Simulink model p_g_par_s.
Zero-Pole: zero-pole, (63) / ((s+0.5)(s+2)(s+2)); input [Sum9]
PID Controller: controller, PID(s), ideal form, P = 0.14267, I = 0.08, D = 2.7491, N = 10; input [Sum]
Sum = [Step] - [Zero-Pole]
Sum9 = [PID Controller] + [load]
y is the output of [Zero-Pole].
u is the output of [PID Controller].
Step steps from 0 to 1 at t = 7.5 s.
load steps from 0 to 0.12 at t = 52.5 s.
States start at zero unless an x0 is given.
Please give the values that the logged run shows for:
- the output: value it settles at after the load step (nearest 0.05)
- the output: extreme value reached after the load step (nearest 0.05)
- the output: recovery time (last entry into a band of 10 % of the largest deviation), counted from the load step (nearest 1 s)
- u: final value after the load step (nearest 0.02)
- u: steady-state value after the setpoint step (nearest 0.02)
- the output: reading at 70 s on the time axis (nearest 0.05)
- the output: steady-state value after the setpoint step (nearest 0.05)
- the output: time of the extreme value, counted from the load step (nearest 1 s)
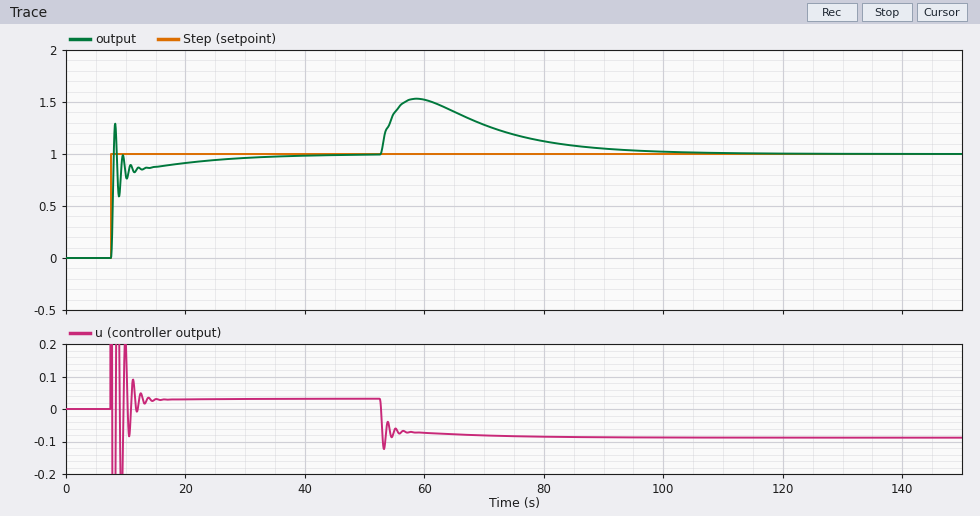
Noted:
1.00
1.55
37 s
-0.08
0.04
1.30
1.00
6 s
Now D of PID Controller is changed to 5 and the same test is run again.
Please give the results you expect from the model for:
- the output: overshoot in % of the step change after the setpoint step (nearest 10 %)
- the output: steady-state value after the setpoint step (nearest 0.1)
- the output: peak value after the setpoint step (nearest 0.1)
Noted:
60 %
1.0
1.6
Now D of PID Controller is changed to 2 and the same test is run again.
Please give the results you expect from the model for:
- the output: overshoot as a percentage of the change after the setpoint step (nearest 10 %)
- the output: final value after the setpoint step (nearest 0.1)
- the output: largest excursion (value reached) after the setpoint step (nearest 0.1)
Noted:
20 %
1.0
1.2
